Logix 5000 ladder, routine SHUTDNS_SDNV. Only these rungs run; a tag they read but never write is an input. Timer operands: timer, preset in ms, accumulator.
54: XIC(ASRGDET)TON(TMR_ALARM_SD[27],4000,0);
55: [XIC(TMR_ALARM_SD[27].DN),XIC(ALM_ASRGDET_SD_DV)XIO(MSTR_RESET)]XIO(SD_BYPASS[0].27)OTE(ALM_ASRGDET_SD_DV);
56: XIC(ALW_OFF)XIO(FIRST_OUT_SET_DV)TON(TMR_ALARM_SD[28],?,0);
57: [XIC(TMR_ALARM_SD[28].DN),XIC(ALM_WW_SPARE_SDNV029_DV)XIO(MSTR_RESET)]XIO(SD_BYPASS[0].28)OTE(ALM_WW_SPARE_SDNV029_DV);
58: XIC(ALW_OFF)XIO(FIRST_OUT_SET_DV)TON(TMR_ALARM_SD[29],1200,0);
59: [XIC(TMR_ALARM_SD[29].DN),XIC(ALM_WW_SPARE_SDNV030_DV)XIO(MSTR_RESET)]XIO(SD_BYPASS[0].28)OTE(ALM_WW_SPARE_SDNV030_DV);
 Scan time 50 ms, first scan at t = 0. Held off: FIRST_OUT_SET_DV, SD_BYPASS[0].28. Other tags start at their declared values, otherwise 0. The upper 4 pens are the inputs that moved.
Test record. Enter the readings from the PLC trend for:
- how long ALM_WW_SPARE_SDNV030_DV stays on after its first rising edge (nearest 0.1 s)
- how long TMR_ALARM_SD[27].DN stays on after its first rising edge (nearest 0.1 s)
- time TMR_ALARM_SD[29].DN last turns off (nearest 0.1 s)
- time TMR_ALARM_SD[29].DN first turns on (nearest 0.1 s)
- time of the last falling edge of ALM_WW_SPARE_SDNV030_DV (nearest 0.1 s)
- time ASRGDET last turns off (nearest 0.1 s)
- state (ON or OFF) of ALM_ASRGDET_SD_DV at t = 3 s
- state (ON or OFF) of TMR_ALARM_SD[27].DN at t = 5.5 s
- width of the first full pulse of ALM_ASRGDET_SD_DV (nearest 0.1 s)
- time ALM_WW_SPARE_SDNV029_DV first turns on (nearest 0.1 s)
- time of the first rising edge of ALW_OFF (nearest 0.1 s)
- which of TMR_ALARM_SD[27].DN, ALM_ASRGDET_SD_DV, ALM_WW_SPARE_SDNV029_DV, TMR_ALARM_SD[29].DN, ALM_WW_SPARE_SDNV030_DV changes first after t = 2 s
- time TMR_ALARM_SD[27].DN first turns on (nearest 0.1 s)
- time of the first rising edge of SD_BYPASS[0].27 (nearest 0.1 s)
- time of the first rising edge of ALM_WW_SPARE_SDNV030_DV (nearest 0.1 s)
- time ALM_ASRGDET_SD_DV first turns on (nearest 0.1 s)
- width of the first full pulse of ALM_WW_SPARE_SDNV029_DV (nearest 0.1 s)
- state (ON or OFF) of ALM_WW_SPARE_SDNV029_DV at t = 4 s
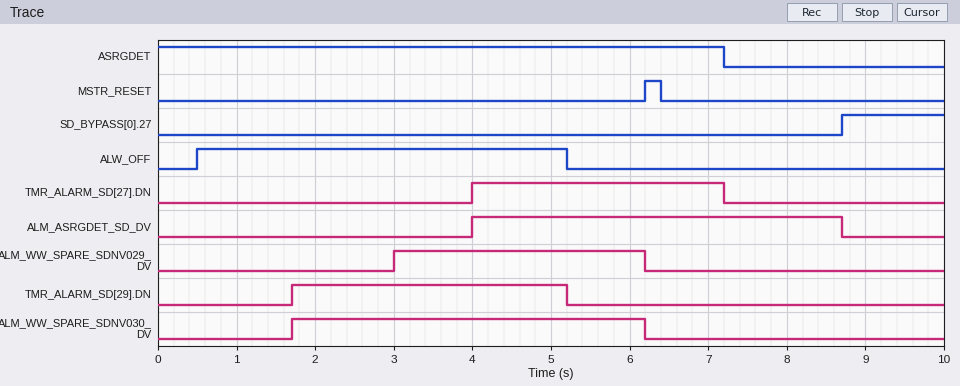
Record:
4.5 s
3.2 s
5.2 s
1.7 s
6.2 s
7.2 s
OFF
ON
4.7 s
3.0 s
0.5 s
ALM_WW_SPARE_SDNV029_DV
4.0 s
8.7 s
1.7 s
4.0 s
3.2 s
ON
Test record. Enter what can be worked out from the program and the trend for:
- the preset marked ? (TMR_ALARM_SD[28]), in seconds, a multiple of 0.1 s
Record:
2.5 s
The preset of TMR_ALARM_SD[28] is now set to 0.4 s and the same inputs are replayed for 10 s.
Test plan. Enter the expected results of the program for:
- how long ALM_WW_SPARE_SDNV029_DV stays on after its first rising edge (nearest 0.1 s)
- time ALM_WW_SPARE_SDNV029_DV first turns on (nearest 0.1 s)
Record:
5.3 s
0.9 s
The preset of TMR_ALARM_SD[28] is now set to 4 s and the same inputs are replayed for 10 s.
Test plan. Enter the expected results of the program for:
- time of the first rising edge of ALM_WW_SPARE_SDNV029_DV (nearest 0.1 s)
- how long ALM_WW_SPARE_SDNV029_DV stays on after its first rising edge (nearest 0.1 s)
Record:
4.5 s
1.7 s
